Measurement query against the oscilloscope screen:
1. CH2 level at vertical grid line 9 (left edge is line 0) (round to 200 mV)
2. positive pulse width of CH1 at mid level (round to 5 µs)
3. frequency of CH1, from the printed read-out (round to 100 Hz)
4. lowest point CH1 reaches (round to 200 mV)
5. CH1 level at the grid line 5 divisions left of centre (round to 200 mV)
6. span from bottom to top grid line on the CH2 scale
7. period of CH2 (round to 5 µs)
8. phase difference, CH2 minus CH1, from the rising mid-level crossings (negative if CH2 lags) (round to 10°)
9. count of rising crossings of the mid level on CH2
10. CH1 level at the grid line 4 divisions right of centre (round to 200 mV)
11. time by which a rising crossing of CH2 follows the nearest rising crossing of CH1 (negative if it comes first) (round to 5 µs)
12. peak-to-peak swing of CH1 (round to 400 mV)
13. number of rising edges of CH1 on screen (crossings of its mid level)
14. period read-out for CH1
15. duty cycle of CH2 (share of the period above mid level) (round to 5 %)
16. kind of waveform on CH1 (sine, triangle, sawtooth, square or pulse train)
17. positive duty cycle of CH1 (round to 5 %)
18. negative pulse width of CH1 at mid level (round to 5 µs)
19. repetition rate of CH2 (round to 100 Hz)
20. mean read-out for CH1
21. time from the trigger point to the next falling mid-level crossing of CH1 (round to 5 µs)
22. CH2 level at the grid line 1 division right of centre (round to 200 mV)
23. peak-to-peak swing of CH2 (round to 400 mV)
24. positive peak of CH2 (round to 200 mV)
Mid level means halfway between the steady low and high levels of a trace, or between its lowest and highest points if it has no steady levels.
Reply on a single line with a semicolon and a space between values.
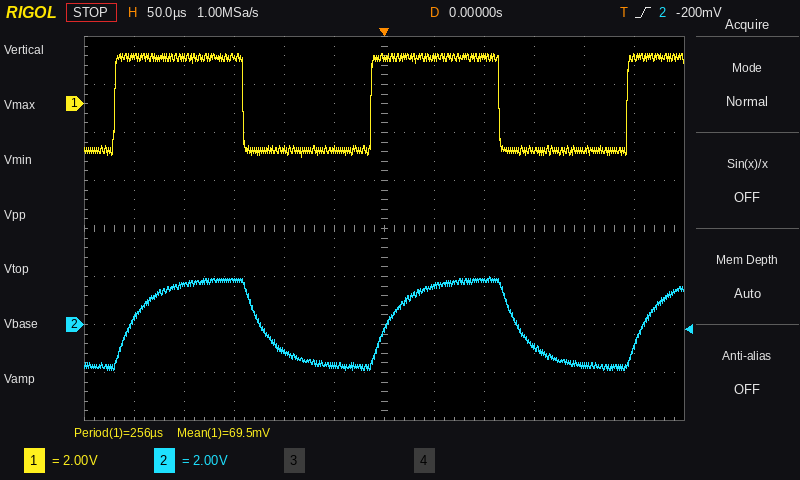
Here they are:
-1.0 V; 130 µs; 3.9 kHz; -2.2 V; 2.0 V; 16 V; 255 µs; -20°; 3; -2.0 V; +15 µs; 4.4 V; 3; 256 µs; 50 %; square; 50 %; 130 µs; 3.9 kHz; 69.5 mV; 115 µs; 1.6 V; 4.0 V; 2.0 V
